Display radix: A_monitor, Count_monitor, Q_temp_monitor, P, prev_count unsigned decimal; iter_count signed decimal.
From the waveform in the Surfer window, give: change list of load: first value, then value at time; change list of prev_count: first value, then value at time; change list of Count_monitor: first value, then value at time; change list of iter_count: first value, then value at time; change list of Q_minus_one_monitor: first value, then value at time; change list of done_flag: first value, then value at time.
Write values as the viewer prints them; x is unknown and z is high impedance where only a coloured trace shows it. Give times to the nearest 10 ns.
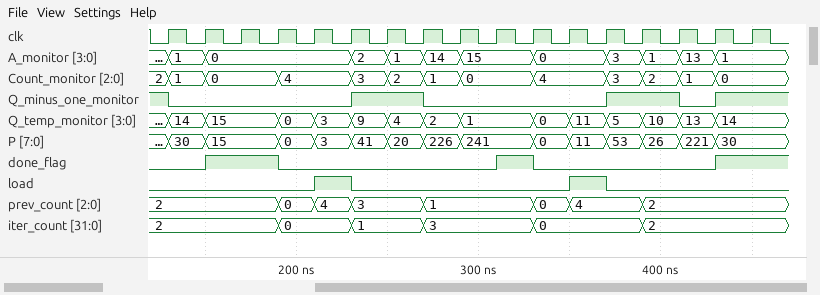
0, 1 at 210 ns, 0 at 230 ns, 1 at 350 ns, 0 at 370 ns
2, 0 at 190 ns, 4 at 210 ns, 3 at 230 ns, 1 at 270 ns, 0 at 330 ns, 4 at 350 ns, 2 at 390 ns
2, 1 at 130 ns, 0 at 150 ns, 4 at 190 ns, 3 at 230 ns, 2 at 250 ns, 1 at 270 ns, 0 at 290 ns, 4 at 330 ns, 3 at 370 ns, 2 at 390 ns, 1 at 410 ns, 0 at 430 ns
2, 0 at 190 ns, 1 at 230 ns, 3 at 270 ns, 0 at 330 ns, 2 at 390 ns
1, 0 at 130 ns, 1 at 230 ns, 0 at 270 ns, 1 at 370 ns, 0 at 410 ns, 1 at 430 ns
0, 1 at 150 ns, 0 at 190 ns, 1 at 310 ns, 0 at 330 ns, 1 at 430 ns
